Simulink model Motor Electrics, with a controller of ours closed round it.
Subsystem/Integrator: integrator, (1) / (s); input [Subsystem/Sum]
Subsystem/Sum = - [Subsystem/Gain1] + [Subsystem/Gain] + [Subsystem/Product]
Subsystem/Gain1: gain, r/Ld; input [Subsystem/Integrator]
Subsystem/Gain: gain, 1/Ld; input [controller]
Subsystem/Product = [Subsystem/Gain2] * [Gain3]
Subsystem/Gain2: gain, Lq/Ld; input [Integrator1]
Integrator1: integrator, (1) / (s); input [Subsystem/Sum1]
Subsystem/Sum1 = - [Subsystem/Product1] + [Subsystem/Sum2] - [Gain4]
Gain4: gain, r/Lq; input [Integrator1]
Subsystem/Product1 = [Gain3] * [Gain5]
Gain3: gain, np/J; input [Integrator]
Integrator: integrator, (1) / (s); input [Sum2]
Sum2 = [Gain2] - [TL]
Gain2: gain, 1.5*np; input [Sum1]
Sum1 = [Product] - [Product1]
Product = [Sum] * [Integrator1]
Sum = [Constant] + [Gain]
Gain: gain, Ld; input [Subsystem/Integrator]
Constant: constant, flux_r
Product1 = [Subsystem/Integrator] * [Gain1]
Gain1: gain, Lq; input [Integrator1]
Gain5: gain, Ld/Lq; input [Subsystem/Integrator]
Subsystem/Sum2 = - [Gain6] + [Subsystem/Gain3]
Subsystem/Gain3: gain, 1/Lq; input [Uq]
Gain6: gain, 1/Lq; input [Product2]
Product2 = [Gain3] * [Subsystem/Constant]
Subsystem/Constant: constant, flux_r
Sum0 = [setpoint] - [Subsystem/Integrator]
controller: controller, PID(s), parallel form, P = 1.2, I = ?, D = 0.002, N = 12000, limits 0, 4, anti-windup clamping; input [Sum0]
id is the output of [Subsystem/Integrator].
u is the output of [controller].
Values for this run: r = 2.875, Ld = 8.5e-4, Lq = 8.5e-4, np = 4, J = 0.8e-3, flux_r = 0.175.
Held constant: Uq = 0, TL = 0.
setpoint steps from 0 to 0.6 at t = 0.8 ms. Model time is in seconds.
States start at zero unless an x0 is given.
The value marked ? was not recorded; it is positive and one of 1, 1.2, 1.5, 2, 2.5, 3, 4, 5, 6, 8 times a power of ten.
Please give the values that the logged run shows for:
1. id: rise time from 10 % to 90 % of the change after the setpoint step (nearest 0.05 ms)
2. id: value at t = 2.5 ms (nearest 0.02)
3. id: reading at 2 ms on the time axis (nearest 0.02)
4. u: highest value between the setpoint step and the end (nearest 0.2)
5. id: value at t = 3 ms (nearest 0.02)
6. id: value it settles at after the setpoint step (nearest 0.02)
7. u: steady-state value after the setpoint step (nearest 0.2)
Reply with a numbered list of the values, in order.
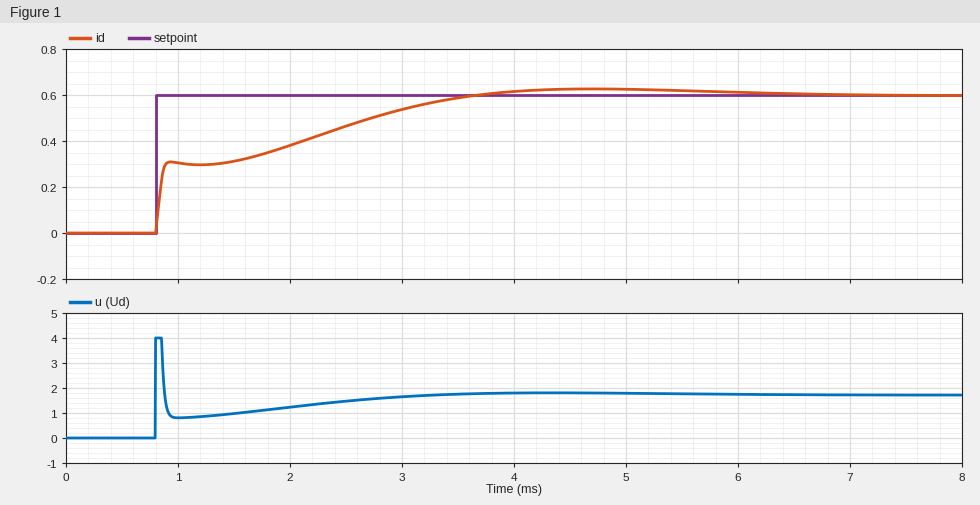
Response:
1. 2.20 ms
2. 0.46
3. 0.38
4. 4.0
5. 0.54
6. 0.60
7. 1.8
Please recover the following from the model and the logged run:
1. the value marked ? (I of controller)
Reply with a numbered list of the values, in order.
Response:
1. 4000
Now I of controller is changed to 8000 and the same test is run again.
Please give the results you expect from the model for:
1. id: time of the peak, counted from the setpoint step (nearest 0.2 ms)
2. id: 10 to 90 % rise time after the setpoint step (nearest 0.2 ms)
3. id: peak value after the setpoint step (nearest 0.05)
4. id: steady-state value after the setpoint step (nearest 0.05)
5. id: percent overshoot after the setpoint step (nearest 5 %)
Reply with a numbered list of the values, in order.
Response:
1. 2.4 ms
2. 1.4 ms
3. 0.65
4. 0.60
5. 10 %
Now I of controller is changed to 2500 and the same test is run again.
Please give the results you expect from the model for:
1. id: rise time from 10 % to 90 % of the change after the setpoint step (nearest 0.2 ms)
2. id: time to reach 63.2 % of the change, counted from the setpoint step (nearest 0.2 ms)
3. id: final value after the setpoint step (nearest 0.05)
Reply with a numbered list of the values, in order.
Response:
1. 3.2 ms
2. 1.6 ms
3. 0.60
